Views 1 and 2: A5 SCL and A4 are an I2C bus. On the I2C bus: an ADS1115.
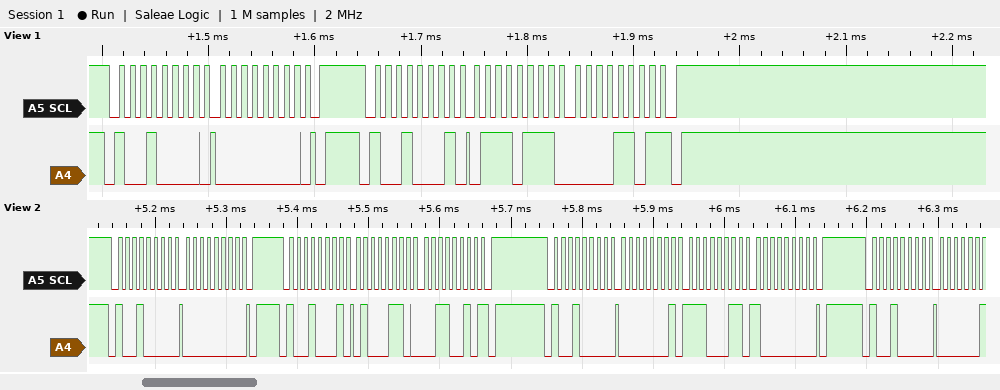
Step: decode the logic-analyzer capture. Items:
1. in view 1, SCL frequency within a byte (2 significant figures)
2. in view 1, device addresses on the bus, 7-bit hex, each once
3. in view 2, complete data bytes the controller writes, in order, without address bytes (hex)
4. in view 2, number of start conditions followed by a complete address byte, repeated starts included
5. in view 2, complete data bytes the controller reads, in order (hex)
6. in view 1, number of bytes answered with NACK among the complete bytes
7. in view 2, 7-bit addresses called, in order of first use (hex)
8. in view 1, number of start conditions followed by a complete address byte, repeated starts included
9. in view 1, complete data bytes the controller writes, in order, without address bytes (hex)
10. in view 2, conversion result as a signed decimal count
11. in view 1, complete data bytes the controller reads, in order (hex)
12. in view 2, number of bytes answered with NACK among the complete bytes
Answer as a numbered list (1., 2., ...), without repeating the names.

1. 100 kHz
2. 0x48
3. 00 01 E3 80
4. 4
5. 46 32
6. 1
7. 0x48
8. 2
9. 00
10. 17970
11. 77 0D
12. 1
